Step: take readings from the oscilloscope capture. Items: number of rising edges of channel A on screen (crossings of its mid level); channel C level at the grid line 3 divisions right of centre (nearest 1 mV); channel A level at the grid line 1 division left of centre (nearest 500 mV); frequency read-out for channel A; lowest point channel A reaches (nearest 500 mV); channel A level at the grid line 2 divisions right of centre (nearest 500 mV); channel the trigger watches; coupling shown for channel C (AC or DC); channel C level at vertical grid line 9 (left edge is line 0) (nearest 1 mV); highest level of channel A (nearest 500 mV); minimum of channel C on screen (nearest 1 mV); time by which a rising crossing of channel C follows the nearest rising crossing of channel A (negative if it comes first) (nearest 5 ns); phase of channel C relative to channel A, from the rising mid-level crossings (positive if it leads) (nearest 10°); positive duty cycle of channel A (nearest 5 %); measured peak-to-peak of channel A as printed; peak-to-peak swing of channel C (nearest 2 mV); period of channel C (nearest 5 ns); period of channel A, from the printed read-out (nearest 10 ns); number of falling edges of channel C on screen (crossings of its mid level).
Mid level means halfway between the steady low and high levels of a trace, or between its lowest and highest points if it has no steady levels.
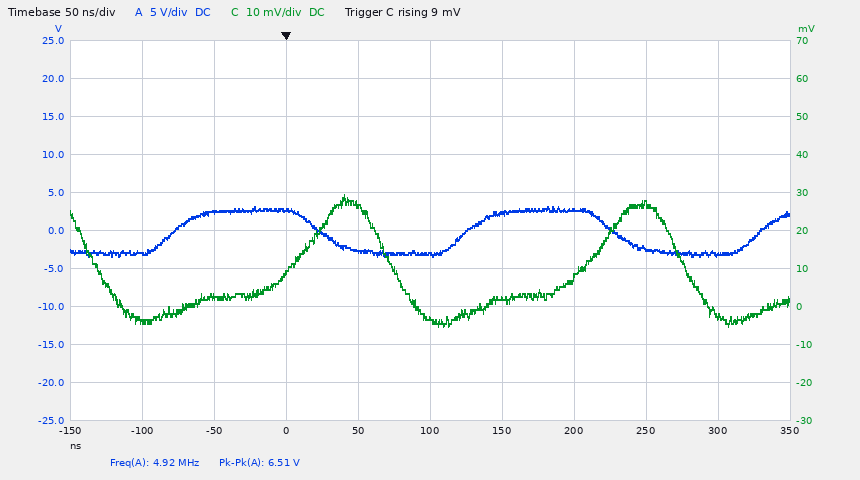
3
27 mV
-2.5 V
4.92 MHz
-3.5 V
3.0 V
channel C
DC
-3 mV
3.0 V
-5 mV
+85 ns
-150°
50 %
6.51 V
34 mV
205 ns
200 ns
3
